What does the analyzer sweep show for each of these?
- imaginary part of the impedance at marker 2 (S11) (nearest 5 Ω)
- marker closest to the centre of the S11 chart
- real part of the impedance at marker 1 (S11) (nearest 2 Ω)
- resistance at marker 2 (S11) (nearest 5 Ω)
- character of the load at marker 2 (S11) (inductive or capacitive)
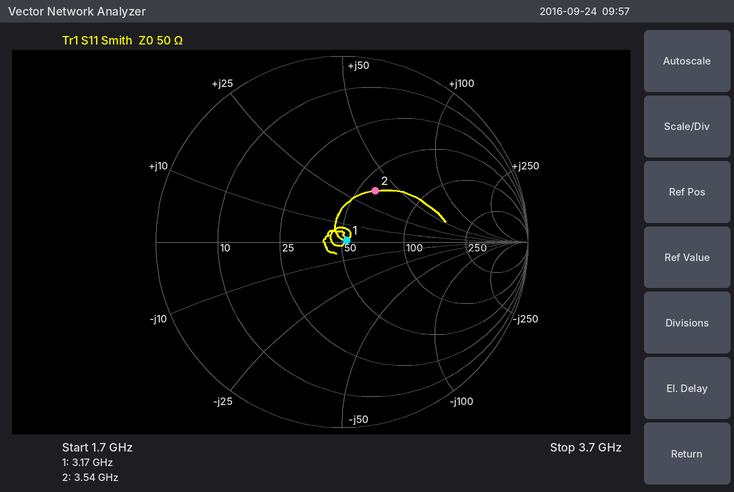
+35 Ω
marker 1
52 Ω
60 Ω
inductive
